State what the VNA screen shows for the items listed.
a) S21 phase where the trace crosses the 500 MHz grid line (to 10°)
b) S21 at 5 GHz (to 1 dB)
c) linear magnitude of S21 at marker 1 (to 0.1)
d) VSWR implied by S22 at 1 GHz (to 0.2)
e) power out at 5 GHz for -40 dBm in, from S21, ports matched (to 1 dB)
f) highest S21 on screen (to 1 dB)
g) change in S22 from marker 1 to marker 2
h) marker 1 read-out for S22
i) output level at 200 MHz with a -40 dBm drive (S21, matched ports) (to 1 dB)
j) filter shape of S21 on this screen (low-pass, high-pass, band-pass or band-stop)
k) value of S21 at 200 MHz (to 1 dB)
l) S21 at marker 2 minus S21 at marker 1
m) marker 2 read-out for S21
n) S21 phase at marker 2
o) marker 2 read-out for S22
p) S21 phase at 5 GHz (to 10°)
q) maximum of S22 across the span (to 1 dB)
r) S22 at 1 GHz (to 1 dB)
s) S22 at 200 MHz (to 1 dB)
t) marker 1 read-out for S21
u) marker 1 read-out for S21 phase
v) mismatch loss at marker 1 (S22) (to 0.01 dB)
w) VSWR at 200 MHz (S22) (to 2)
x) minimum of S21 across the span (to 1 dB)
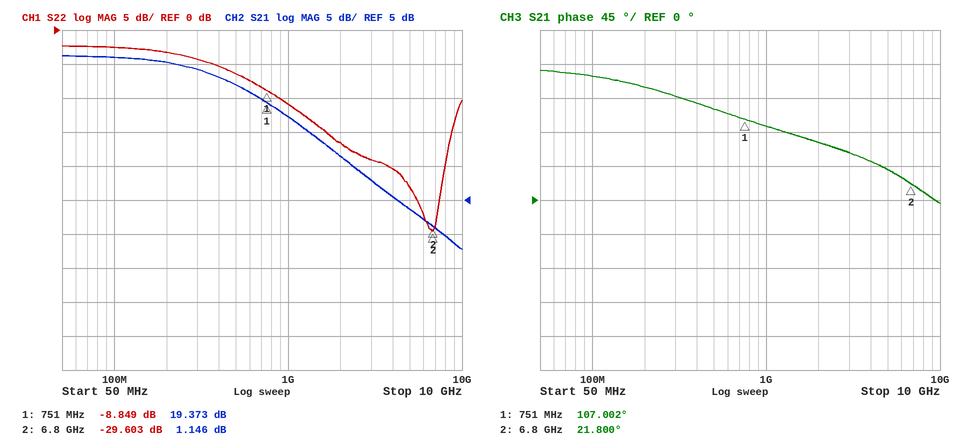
120°
4 dB
9.3
1.8
-36 dBm
26 dB
-20.754 dB
-8.849 dB
-15 dBm
low-pass
25 dB
-18.227 dB
1.146 dB
21.800°
-29.603 dB
40°
-2 dB
-11 dB
-3 dB
19.373 dB
107.002°
0.61 dB
6
-2 dB
